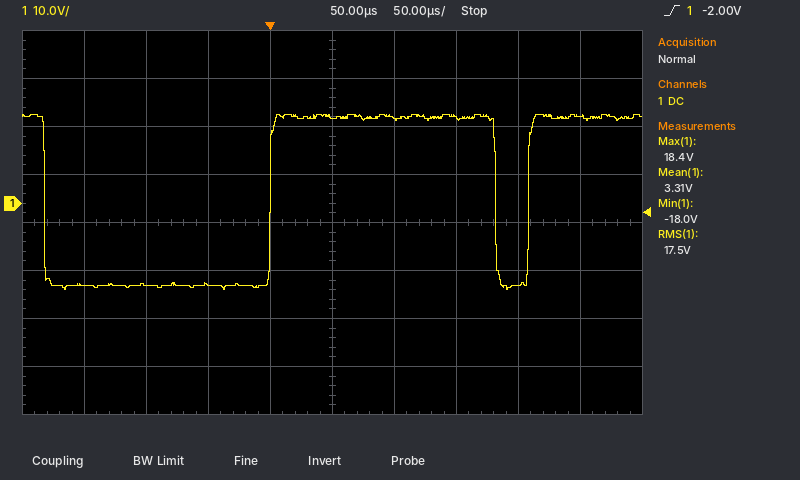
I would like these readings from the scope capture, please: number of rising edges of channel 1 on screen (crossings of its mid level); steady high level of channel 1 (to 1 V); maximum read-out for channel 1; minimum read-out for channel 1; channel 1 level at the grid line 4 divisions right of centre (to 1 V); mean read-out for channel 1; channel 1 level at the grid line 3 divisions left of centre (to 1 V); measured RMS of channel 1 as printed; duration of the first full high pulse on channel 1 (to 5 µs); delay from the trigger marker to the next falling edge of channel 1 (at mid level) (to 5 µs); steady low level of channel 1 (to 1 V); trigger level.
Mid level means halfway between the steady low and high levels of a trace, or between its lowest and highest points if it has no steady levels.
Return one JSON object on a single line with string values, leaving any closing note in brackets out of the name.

{"number of rising edges of channel 1 on screen": "2", "steady high level of channel 1": "18 V", "maximum read-out for channel 1": "18.4 V", "minimum read-out for channel 1": "-18.0 V", "channel 1 level at the grid line 4 divisions right of centre": "18 V", "mean read-out for channel 1": "3.31 V", "channel 1 level at the grid line 3 divisions left of centre": "-17 V", "measured RMS of channel 1 as printed": "17.5 V", "duration of the first full high pulse on channel 1": "180 µs", "delay from the trigger marker to the next falling edge of channel 1 (at mid level)": "180 µs", "steady low level of channel 1": "-17 V", "trigger level": "-2.00 V"}
